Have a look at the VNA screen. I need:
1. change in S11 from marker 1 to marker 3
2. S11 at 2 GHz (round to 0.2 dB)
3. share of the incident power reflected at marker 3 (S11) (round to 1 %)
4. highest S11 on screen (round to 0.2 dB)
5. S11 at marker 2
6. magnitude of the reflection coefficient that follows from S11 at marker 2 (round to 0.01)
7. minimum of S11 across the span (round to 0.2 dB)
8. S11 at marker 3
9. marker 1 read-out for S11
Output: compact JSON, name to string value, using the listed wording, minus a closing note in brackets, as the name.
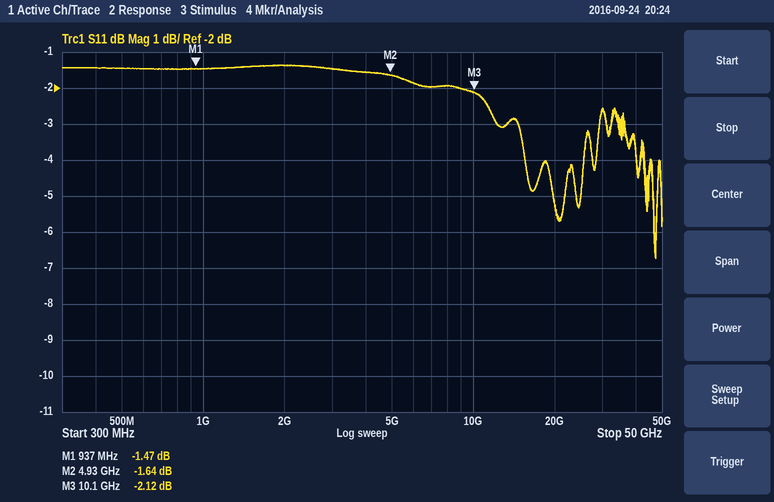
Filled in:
{"change in S11 from marker 1 to marker 3": "-0.65 dB", "S11 at 2 GHz": "-1.4 dB", "share of the incident power reflected at marker 3 (S11)": "61 %", "highest S11 on screen": "-1.4 dB", "S11 at marker 2": "-1.64 dB", "magnitude of the reflection coefficient that follows from S11 at marker 2": "0.83", "minimum of S11 across the span": "-6.8 dB", "S11 at marker 3": "-2.12 dB", "marker 1 read-out for S11": "-1.47 dB"}
